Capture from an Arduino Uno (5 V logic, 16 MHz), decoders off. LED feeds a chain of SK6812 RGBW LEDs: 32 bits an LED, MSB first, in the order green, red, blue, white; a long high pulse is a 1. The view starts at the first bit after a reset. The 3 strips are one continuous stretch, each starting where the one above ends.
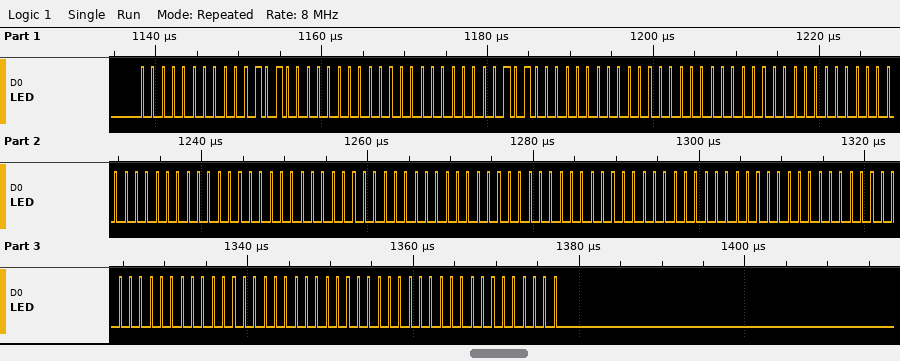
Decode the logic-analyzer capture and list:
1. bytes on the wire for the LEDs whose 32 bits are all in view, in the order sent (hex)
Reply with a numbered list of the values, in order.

1. 00 14 00 00 14 00 00 00 00 00 00 00 00 00 00 00 00 00 00 00 00 00 00 00
